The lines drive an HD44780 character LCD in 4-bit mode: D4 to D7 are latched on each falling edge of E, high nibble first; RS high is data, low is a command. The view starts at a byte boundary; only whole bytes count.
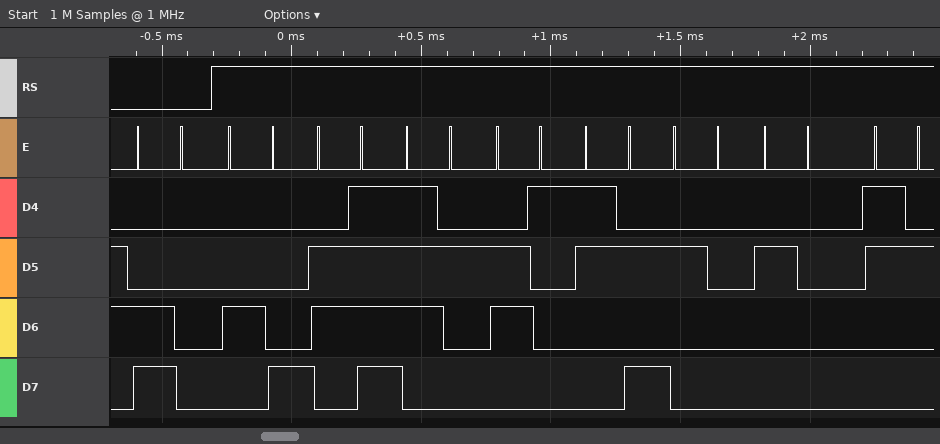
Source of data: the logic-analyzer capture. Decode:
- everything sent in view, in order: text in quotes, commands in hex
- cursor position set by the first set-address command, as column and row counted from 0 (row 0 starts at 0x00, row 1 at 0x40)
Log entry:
0xC0 "Hora:  2"
column 0, row 1
